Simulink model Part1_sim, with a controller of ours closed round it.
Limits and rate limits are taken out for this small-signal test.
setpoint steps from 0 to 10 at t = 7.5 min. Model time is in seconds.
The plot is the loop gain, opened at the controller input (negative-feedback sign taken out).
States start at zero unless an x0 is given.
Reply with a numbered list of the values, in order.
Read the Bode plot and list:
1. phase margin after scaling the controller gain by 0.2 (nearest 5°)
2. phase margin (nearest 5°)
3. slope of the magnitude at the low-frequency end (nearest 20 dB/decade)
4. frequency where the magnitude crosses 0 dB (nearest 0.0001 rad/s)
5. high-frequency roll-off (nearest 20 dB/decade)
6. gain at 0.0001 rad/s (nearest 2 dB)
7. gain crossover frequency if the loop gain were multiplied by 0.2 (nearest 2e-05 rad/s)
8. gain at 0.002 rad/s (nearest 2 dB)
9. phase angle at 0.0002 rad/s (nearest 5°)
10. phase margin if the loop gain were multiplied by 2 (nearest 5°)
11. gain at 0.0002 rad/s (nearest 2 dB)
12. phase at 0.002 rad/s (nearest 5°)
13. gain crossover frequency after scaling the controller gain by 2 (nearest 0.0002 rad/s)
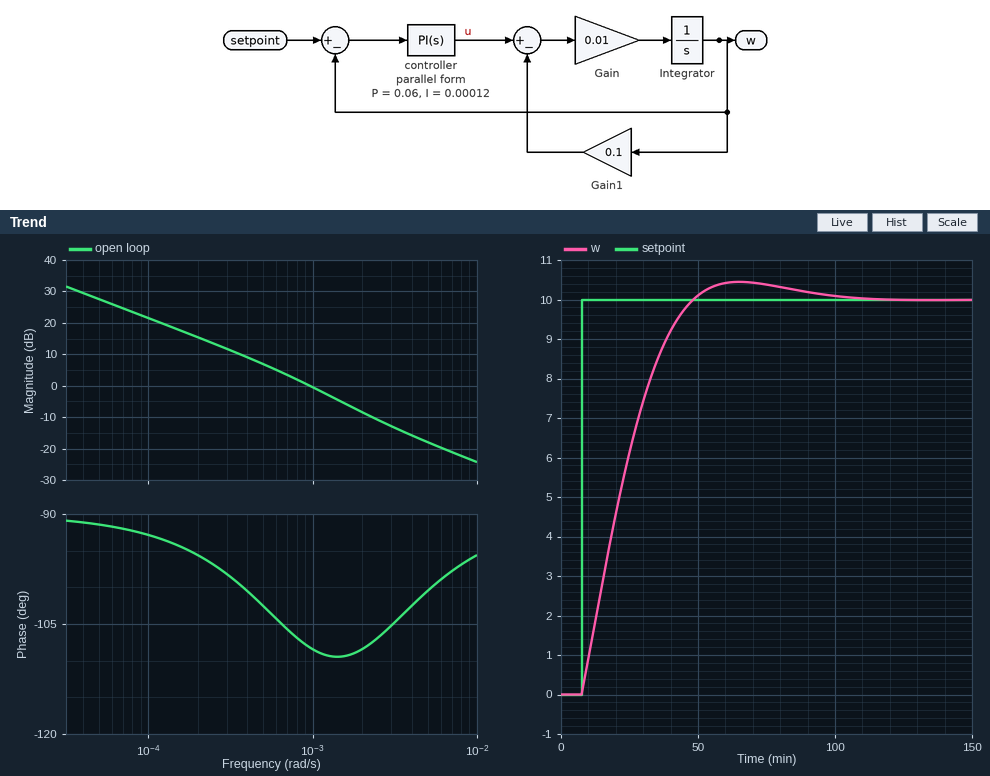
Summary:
1. 85°
2. 70°
3. -20 dB/decade
4. 0.0010 rad/s
5. -20 dB/decade
6. 22 dB
7. 0.00024 rad/s
8. -8 dB
9. -95°
10. 70°
11. 16 dB
12. -110°
13. 0.0016 rad/s
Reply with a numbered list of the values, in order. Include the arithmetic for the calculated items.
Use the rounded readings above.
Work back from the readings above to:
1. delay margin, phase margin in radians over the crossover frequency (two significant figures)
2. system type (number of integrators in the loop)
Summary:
1. 70 × π / 180 / 0.001 = 1200 s
2. 1
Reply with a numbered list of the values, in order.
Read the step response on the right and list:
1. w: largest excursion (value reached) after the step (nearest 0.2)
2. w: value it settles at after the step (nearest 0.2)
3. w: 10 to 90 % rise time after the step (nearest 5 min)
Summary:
1. 10.4
2. 10.0
3. 30 min
